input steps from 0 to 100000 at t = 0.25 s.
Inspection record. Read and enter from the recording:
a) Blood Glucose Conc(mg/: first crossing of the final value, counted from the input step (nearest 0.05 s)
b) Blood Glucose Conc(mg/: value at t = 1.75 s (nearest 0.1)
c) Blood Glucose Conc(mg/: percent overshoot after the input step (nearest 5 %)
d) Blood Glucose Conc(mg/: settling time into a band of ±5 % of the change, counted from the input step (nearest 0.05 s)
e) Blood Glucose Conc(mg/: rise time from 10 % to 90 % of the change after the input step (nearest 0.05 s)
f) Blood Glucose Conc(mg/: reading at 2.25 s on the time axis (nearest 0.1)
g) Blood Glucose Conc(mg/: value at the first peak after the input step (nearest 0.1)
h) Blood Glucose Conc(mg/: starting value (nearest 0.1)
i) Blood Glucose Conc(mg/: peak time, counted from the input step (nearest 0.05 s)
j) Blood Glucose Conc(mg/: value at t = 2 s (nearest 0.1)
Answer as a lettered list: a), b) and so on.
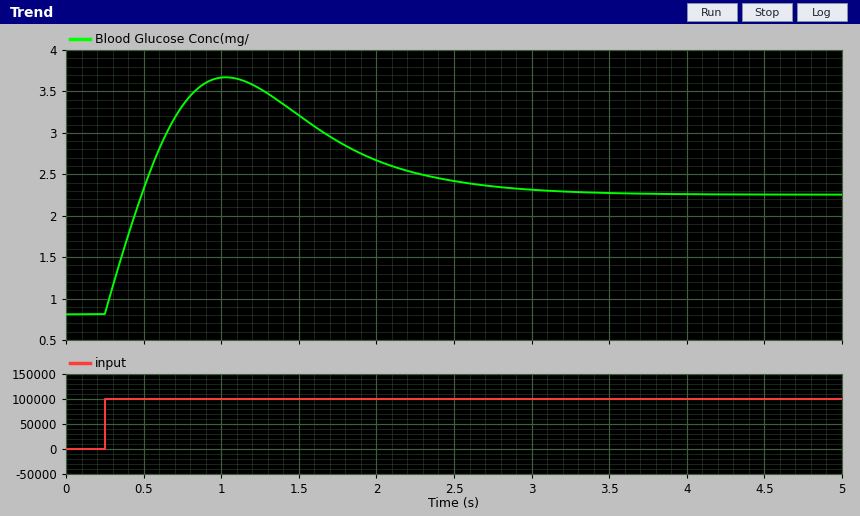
a) 0.25 s
b) 2.9
c) 100 %
d) 2.65 s
e) 0.20 s
f) 2.5
g) 3.7
h) 0.8
i) 0.80 s
j) 2.7
